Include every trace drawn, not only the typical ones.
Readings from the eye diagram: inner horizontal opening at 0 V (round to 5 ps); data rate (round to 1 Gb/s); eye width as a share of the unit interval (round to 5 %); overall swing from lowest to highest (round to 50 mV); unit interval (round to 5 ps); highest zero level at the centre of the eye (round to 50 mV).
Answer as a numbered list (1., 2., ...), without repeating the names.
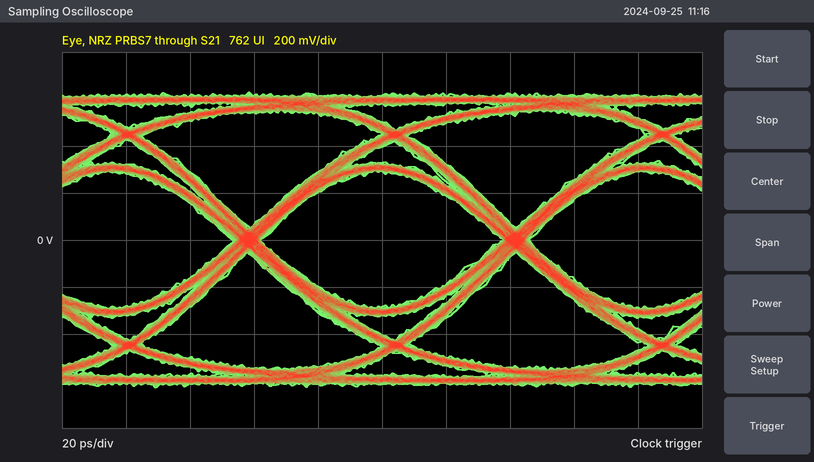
1. 75 ps
2. 12 Gb/s
3. 90 %
4. 1.25 V
5. 85 ps
6. -300 mV
